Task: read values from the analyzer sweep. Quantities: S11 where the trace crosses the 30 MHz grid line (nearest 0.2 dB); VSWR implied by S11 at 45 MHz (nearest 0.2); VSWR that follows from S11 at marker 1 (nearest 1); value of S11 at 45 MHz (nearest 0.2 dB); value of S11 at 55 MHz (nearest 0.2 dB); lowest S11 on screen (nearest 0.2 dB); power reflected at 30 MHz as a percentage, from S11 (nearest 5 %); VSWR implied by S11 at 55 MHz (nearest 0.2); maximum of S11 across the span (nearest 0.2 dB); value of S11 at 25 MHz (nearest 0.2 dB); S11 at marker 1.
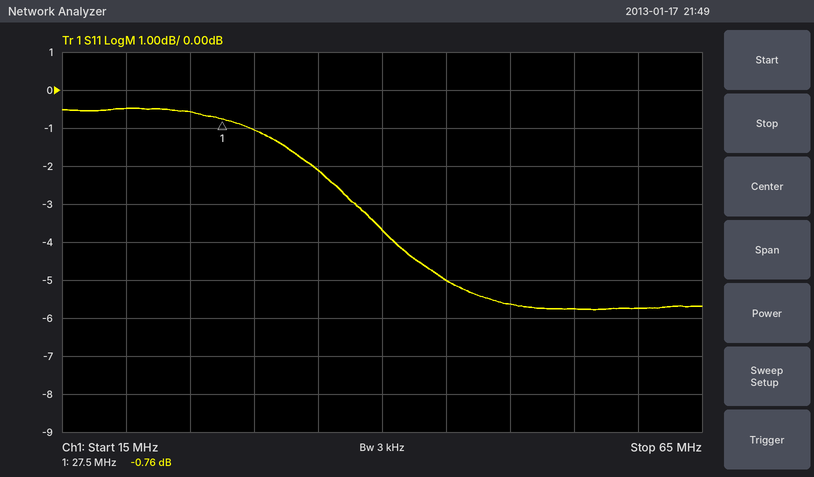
-1.0 dB
3.6
23
-5.0 dB
-5.8 dB
-5.8 dB
80 %
3.2
-0.4 dB
-0.6 dB
-0.76 dB
